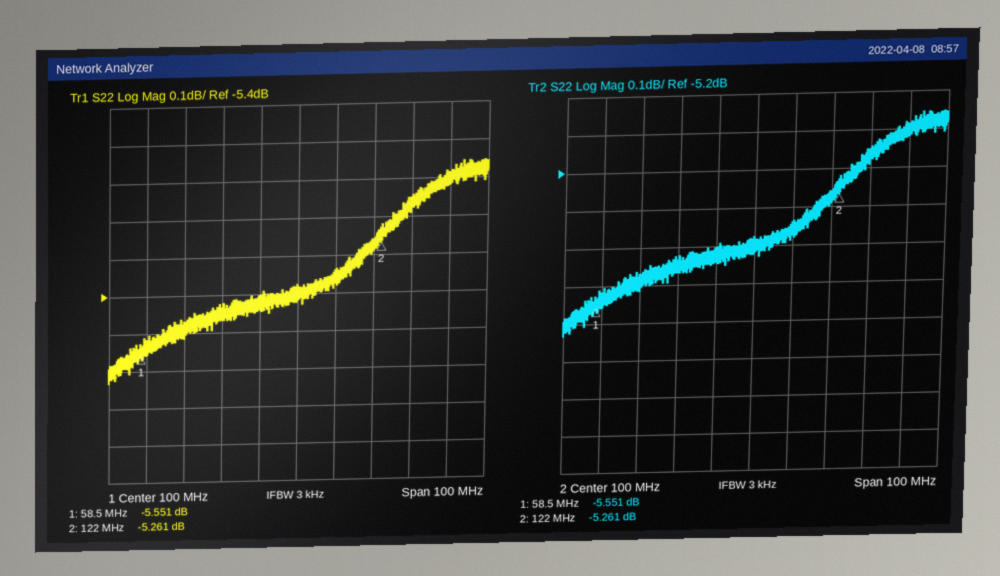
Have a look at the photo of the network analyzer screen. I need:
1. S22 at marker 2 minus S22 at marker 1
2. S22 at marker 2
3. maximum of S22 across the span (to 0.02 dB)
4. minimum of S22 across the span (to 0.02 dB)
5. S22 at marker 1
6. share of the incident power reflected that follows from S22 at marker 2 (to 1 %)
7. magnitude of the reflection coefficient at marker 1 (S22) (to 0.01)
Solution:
0.290 dB
-5.261 dB
-5.06 dB
-5.64 dB
-5.551 dB
30 %
0.53
